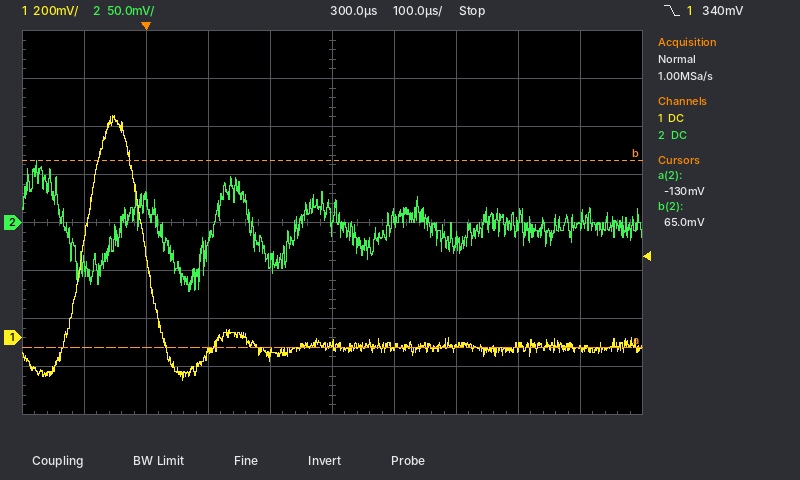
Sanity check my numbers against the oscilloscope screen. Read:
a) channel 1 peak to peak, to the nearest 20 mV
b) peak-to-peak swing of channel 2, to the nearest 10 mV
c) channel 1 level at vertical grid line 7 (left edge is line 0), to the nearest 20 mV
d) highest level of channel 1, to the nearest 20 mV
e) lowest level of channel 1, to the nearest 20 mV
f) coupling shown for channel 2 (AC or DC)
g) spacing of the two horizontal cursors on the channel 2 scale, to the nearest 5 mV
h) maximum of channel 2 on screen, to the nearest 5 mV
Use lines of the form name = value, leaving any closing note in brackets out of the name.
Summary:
channel 1 peak to peak, to the nearest 20 mV = 1.10 V
peak-to-peak swing of channel 2, to the nearest 10 mV = 140 mV
channel 1 level at vertical grid line 7 (left edge is line 0), to the nearest 20 mV = -40 mV
highest level of channel 1, to the nearest 20 mV = 920 mV
lowest level of channel 1, to the nearest 20 mV = -180 mV
coupling shown for channel 2 = DC
spacing of the two horizontal cursors on the channel 2 scale, to the nearest 5 mV = 195 mV
maximum of channel 2 on screen, to the nearest 5 mV = 65 mV
